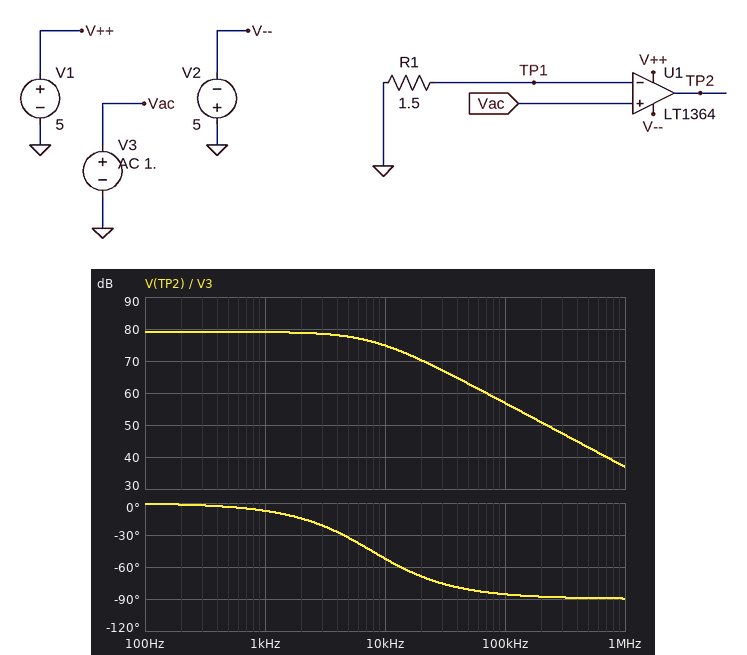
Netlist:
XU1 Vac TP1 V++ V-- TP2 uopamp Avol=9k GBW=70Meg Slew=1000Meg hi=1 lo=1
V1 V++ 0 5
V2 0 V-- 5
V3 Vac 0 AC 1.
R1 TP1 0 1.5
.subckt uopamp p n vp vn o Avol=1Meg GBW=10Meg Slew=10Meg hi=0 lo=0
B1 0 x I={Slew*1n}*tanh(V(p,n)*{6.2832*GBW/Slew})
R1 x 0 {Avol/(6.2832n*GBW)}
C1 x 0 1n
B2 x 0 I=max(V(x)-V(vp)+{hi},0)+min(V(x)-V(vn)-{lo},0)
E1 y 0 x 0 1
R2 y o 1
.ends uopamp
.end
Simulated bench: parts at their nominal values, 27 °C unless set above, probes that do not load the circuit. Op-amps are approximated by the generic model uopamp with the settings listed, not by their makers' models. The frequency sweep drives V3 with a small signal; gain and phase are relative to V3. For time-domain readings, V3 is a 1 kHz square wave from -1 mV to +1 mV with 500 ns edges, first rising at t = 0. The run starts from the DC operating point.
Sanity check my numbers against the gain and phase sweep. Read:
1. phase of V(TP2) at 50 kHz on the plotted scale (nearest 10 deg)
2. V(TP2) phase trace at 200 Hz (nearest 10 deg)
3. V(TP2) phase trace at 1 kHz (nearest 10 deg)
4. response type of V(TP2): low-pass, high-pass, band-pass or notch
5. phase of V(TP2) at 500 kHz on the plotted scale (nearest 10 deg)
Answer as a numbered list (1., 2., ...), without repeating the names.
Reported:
1. -80 deg
2. 0 deg
3. -10 deg
4. low-pass
5. -90 deg
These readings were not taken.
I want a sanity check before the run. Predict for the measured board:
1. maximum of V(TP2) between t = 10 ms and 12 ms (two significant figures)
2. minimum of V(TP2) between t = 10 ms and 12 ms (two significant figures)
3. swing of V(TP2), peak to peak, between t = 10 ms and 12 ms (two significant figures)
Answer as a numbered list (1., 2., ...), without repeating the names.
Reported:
1. 4.0 V
2. -4.0 V
3. 8.0 V
